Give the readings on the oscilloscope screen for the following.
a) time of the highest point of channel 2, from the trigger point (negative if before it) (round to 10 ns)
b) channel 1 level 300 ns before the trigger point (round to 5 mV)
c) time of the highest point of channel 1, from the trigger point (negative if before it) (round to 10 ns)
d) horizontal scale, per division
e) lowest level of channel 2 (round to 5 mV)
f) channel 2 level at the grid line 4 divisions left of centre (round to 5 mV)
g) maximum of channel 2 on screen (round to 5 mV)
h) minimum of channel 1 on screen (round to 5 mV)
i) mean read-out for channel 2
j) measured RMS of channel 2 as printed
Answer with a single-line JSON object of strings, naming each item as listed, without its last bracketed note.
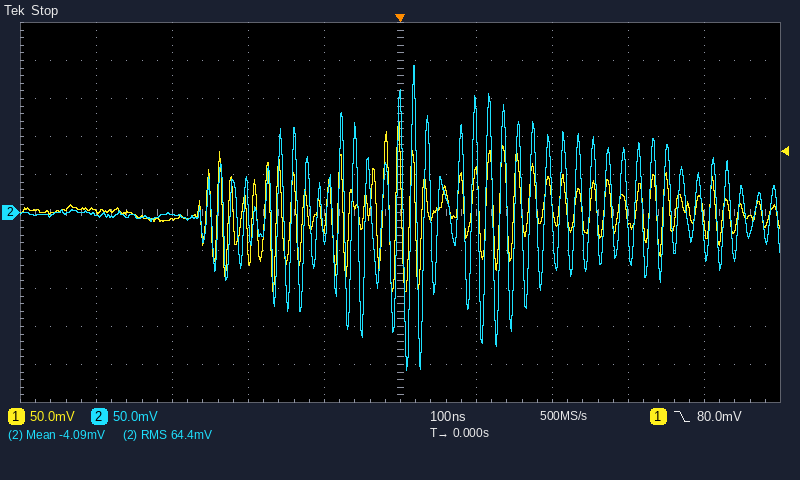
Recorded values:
{"time of the highest point of channel 2, from the trigger point (negative if before it)": "+20 ns", "channel 1 level 300 ns before the trigger point": "-10 mV", "time of the highest point of channel 1, from the trigger point (negative if before it)": "0 ns", "horizontal scale, per division": "100 ns", "lowest level of channel 2": "-210 mV", "channel 2 level at the grid line 4 divisions left of centre": "-5 mV", "maximum of channel 2 on screen": "195 mV", "minimum of channel 1 on screen": "-105 mV", "mean read-out for channel 2": "-4.09 mV", "measured RMS of channel 2 as printed": "64.4 mV"}
